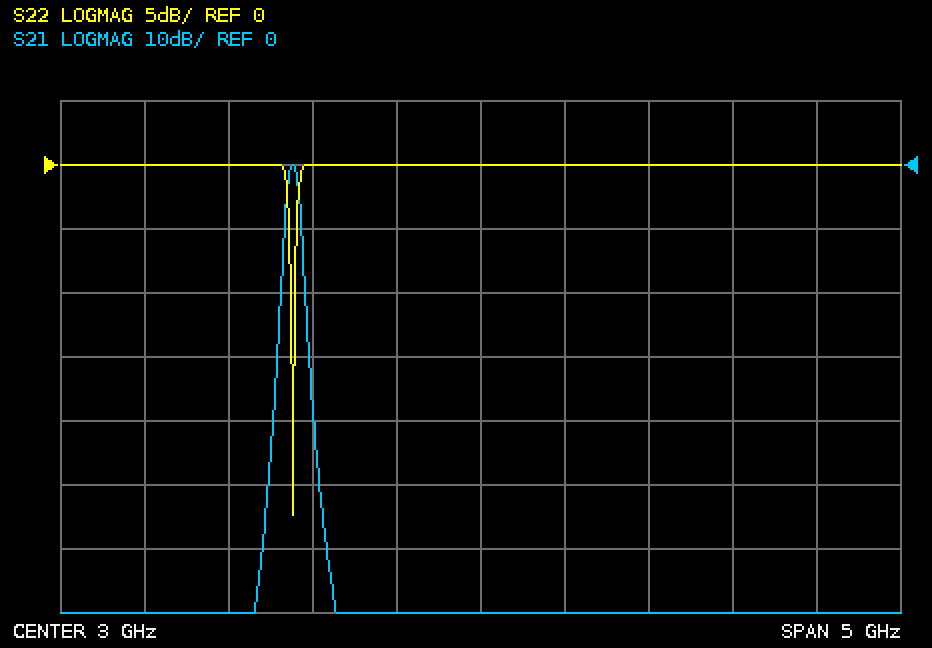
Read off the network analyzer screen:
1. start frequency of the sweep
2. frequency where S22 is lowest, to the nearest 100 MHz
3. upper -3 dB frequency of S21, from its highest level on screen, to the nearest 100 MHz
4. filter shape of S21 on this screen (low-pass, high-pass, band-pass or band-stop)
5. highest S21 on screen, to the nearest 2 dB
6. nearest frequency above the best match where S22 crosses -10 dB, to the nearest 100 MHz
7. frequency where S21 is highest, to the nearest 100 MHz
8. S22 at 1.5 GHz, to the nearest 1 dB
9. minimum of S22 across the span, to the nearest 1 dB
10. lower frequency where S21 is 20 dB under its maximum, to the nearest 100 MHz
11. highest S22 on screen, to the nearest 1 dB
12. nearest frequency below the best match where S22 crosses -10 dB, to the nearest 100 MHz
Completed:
500 MHz
1.9 GHz
1.9 GHz
band-pass
0 dB
1.9 GHz
1.9 GHz
0 dB
-27 dB
1.8 GHz
0 dB
1.9 GHz
